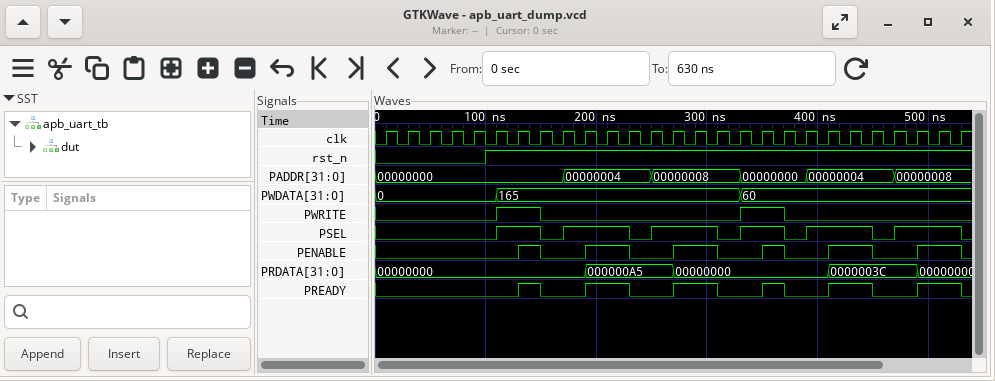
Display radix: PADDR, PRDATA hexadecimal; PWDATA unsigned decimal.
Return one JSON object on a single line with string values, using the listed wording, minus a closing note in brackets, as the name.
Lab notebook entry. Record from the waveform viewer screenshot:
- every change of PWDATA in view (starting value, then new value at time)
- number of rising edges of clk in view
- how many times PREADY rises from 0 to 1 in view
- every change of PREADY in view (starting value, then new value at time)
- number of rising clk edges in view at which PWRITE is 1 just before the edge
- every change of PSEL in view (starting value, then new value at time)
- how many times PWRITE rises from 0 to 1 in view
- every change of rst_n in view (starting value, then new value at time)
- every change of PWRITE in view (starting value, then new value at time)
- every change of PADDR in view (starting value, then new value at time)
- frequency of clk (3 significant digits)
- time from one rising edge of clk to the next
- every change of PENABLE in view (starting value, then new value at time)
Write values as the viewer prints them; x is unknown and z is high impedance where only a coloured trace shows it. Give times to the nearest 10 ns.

{"every change of PWDATA in view": "0, 165 at 110 ns, 60 at 330 ns", "number of rising edges of clk in view": "27", "how many times PREADY rises from 0 to 1 in view": "6", "every change of PREADY in view": "0, 1 at 130 ns, 0 at 150 ns, 1 at 190 ns, 0 at 230 ns, 1 at 270 ns, 0 at 310 ns, 1 at 350 ns, 0 at 370 ns, 1 at 410 ns, 0 at 450 ns, 1 at 490 ns, 0 at 530 ns", "number of rising clk edges in view at which PWRITE is 1 just before the edge": "4", "every change of PSEL in view": "0, 1 at 110 ns, 0 at 150 ns, 1 at 170 ns, 0 at 230 ns, 1 at 250 ns, 0 at 310 ns, 1 at 330 ns, 0 at 370 ns, 1 at 390 ns, 0 at 450 ns, 1 at 470 ns, 0 at 530 ns", "how many times PWRITE rises from 0 to 1 in view": "2", "every change of rst_n in view": "0, 1 at 100 ns", "every change of PWRITE in view": "0, 1 at 110 ns, 0 at 150 ns, 1 at 330 ns, 0 at 370 ns", "every change of PADDR in view": "00000000, 00000004 at 170 ns, 00000008 at 250 ns, 00000000 at 330 ns, 00000004 at 390 ns, 00000008 at 470 ns", "frequency of clk": "50.0 MHz", "time from one rising edge of clk to the next": "20 ns", "every change of PENABLE in view": "0, 1 at 130 ns, 0 at 150 ns, 1 at 190 ns, 0 at 230 ns, 1 at 270 ns, 0 at 310 ns, 1 at 350 ns, 0 at 370 ns, 1 at 410 ns, 0 at 450 ns, 1 at 490 ns, 0 at 530 ns"}
